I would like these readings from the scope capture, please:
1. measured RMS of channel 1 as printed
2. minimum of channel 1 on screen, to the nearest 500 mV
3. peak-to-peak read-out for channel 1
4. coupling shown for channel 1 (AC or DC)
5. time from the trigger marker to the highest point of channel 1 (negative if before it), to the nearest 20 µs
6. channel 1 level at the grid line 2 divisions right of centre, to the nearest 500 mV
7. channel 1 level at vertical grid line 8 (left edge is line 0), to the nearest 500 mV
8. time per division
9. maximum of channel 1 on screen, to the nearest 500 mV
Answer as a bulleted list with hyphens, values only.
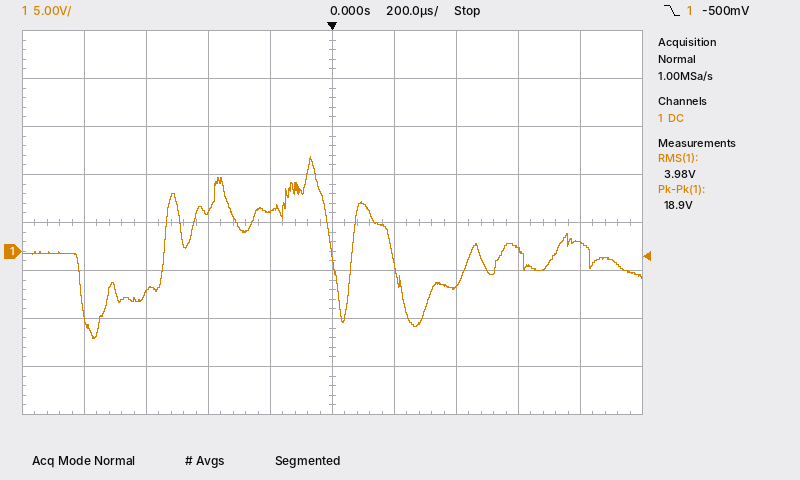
- 3.98 V
- -9.0 V
- 18.9 V
- DC
- -60 µs
- -3.5 V
- 0.0 V
- 200 µs
- 10.0 V
